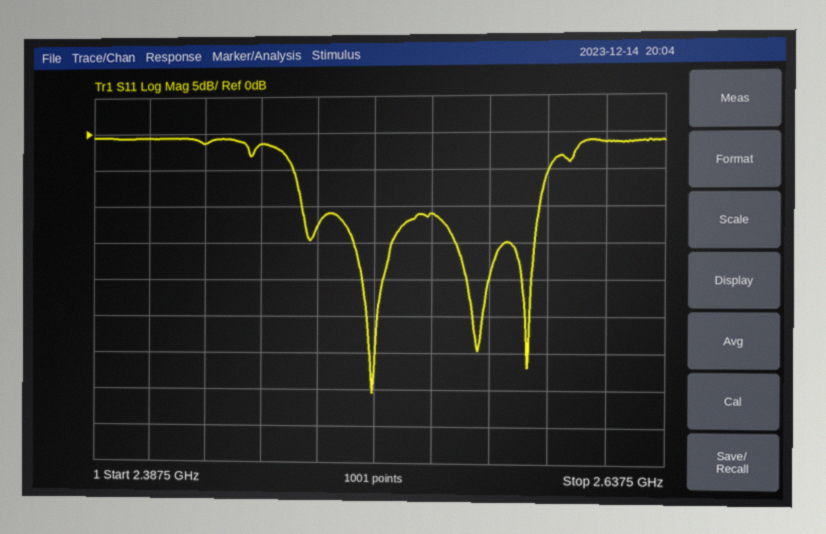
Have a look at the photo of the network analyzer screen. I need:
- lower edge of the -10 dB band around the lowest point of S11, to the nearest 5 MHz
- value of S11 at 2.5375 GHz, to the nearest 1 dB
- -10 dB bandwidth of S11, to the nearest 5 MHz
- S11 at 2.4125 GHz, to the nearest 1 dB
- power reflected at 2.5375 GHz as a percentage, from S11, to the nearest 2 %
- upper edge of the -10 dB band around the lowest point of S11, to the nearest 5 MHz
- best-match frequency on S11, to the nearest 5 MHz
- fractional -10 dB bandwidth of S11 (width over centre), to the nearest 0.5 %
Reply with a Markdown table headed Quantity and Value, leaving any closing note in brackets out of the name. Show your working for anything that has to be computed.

| Quantity | Value |
|---|---|
| lower edge of the -10 dB band around the lowest point of S11, to the nearest 5 MHz | 2.480 GHz |
| value of S11 at 2.5375 GHz, to the nearest 1 dB | -11 dB |
| -10 dB bandwidth of S11, to the nearest 5 MHz | 2.585 GHz − 2.480 GHz = 105 MHz |
| S11 at 2.4125 GHz, to the nearest 1 dB | -1 dB |
| power reflected at 2.5375 GHz as a percentage, from S11, to the nearest 2 % | 10^(-11/10) ≈ 8 % |
| upper edge of the -10 dB band around the lowest point of S11, to the nearest 5 MHz | 2.585 GHz |
| best-match frequency on S11, to the nearest 5 MHz | 2.510 GHz |
| fractional -10 dB bandwidth of S11 (width over centre), to the nearest 0.5 % | 105 MHz / 2.5325 GHz ≈ 4.15 %, so 4.0 % to the nearest 0.5 % |
